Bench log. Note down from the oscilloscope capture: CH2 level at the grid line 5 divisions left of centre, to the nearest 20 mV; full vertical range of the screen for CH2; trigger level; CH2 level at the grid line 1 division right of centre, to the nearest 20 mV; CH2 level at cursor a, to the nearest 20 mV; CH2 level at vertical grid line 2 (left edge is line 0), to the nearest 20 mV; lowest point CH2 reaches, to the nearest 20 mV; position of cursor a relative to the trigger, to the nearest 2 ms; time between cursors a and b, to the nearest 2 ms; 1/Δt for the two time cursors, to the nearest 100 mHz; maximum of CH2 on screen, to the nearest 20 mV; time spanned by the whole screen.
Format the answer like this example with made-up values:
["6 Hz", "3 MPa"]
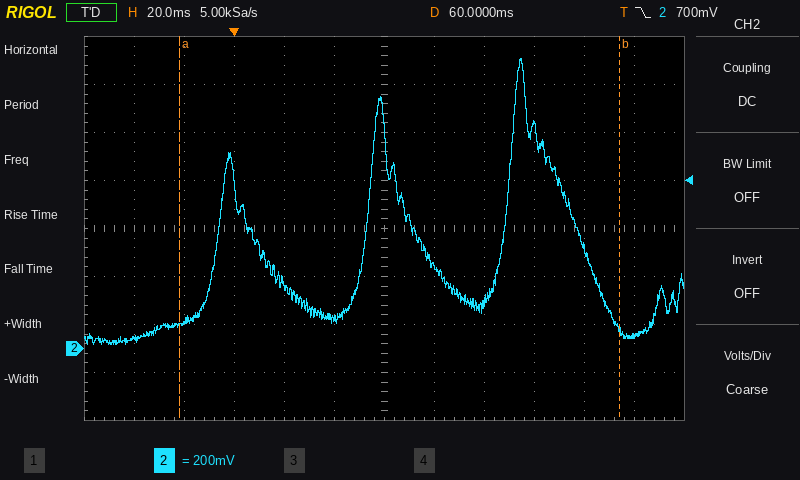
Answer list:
["40 mV", "1.6 V", "700 mV", "340 mV", "100 mV", "120 mV", "20 mV", "-22 ms", "176 ms", "5.7 Hz", "1.20 V", "240 ms"]
